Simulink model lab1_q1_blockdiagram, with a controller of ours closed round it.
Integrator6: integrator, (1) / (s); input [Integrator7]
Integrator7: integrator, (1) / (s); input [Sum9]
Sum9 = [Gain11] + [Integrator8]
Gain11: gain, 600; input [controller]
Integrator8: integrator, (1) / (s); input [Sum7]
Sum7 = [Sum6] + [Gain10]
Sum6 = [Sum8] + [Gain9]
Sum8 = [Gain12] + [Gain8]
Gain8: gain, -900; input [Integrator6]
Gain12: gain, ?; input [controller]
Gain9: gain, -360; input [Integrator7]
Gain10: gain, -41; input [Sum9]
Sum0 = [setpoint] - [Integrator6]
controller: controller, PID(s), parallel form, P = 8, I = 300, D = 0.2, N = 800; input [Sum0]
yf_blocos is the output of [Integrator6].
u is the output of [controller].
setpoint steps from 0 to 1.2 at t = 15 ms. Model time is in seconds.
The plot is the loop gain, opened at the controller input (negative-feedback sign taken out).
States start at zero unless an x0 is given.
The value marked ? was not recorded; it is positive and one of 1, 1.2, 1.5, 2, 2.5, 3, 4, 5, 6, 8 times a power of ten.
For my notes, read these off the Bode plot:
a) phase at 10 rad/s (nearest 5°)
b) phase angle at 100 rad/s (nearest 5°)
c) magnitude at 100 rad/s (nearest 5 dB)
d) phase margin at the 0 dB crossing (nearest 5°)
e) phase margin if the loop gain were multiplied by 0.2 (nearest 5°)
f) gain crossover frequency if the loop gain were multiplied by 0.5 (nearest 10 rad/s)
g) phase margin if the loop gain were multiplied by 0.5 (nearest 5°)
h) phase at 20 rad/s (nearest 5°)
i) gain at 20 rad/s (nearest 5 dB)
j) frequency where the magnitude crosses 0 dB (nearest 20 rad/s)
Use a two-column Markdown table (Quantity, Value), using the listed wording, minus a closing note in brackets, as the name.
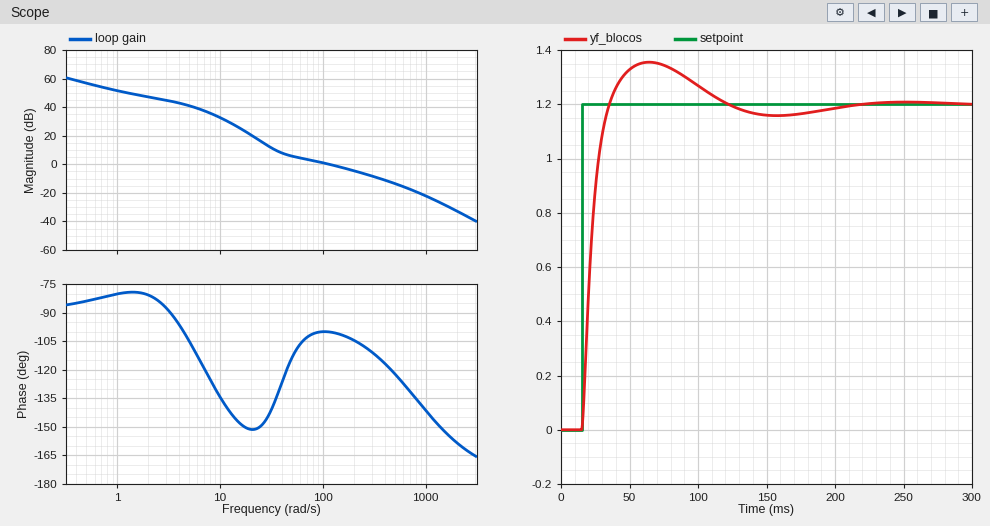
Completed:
| Quantity | Value |
|---|---|
| phase at 10 rad/s | -135° |
| phase angle at 100 rad/s | -100° |
| magnitude at 100 rad/s | 0 dB |
| phase margin at the 0 dB crossing | 80° |
| phase margin if the loop gain were multiplied by 0.2 | 35° |
| gain crossover frequency if the loop gain were multiplied by 0.5 | 50 rad/s |
| phase margin if the loop gain were multiplied by 0.5 | 65° |
| phase at 20 rad/s | -150° |
| gain at 20 rad/s | 20 dB |
| frequency where the magnitude crosses 0 dB | 120 rad/s |
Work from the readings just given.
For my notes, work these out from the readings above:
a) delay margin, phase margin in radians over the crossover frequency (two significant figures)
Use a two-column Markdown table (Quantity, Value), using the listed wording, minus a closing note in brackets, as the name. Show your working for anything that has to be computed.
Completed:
| Quantity | Value |
|---|---|
| delay margin, phase margin in radians over the crossover frequency | 80 × π / 180 / 120 = 0.012 s |
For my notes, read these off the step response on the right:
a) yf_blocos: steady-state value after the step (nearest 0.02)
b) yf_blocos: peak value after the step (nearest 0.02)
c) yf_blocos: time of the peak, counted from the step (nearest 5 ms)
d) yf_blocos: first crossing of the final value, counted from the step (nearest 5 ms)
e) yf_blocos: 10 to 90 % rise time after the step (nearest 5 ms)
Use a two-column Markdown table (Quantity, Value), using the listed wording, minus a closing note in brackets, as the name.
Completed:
| Quantity | Value |
|---|---|
| yf_blocos: steady-state value after the step | 1.20 |
| yf_blocos: peak value after the step | 1.36 |
| yf_blocos: time of the peak, counted from the step | 50 ms |
| yf_blocos: first crossing of the final value, counted from the step | 20 ms |
| yf_blocos: 10 to 90 % rise time after the step | 15 ms |
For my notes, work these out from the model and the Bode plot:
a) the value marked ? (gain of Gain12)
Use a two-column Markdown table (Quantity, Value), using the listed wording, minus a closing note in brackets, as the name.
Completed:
| Quantity | Value |
|---|---|
| the value marked ? | 1000 |
